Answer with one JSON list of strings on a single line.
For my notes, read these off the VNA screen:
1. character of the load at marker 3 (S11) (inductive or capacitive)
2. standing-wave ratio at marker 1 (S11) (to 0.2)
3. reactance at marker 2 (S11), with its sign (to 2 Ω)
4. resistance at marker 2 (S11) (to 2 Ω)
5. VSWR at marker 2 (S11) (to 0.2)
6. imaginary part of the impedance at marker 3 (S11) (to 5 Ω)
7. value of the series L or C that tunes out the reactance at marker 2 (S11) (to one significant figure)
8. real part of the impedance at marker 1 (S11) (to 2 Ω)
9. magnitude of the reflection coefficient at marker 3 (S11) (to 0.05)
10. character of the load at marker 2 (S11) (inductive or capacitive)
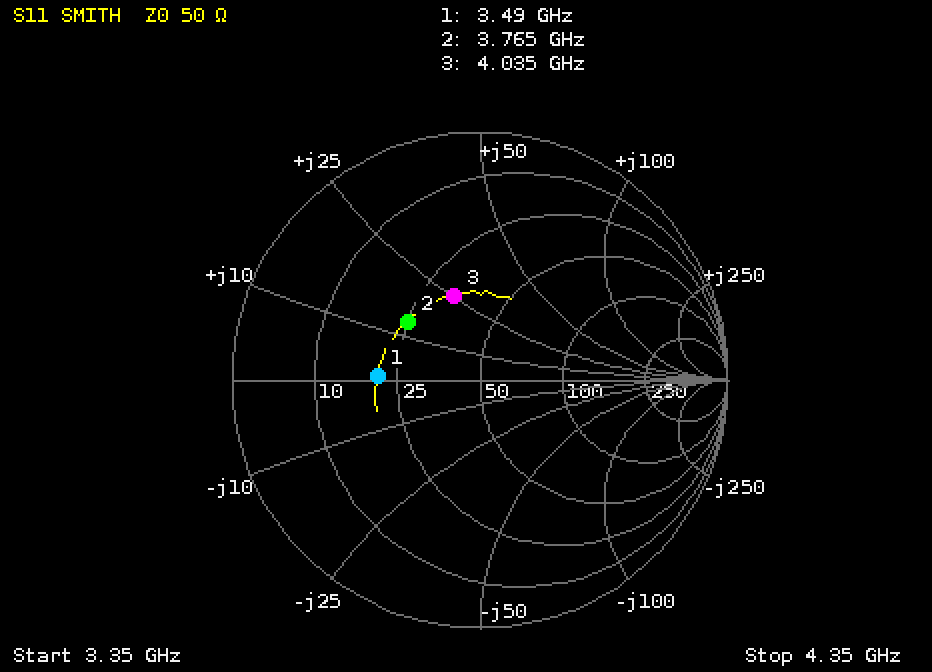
["inductive", "2.4", "+14 Ω", "24 Ω", "2.2", "+25 Ω", "3 pF", "20 Ω", "0.35", "inductive"]
